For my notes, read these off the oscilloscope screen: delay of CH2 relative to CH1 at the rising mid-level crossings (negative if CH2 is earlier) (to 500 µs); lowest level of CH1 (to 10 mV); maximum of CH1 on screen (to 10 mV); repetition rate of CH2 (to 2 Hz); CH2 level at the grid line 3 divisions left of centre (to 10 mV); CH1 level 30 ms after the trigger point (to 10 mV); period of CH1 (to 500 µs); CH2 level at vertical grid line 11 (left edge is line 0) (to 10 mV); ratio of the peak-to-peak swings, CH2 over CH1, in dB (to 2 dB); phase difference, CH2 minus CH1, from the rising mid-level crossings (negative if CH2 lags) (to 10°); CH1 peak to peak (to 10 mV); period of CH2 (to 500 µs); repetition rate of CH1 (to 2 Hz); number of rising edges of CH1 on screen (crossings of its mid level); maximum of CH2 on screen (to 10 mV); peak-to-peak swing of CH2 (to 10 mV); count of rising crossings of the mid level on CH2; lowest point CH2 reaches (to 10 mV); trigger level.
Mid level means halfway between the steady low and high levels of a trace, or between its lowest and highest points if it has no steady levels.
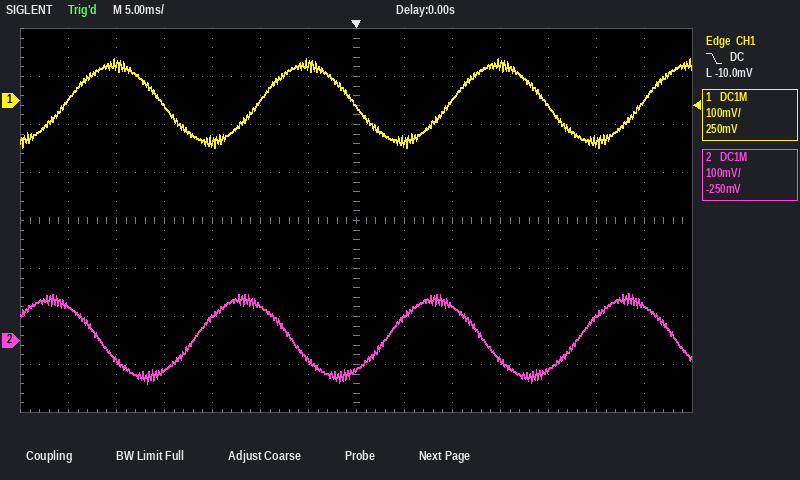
-6.5 ms
-100 mV
90 mV
50 Hz
50 mV
0 mV
20.0 ms
-60 mV
0 dB
+120°
190 mV
20.0 ms
50 Hz
4
100 mV
190 mV
3
-90 mV
-10.0 mV
